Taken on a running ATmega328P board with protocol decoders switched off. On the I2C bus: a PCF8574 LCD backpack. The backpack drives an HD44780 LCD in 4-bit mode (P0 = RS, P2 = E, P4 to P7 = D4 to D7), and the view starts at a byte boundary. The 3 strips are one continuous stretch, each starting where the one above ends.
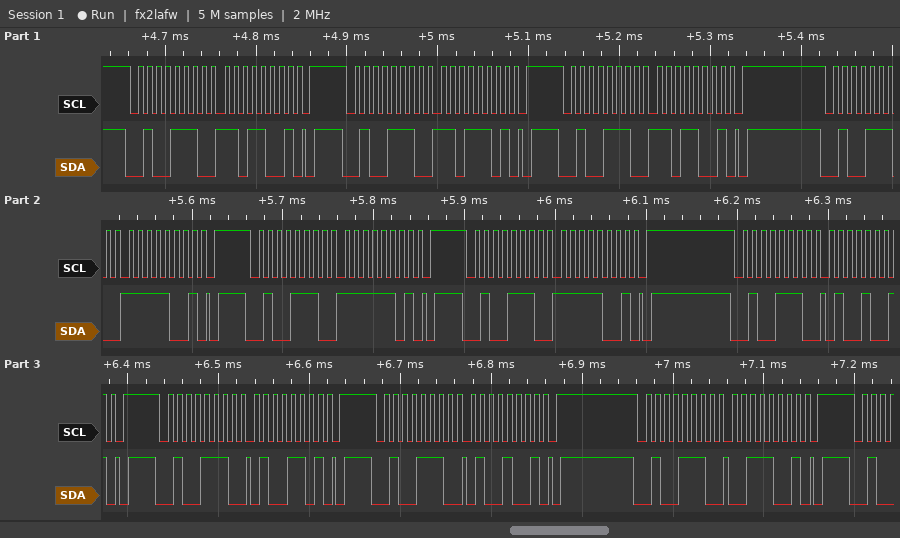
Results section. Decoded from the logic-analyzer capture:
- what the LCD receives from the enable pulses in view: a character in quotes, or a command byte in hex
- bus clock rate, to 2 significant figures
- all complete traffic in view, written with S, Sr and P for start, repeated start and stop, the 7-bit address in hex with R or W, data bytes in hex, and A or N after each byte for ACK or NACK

data 0xDF
100 kHz
S 27W A D9 A P S 27W A DD A P S 27W A D9 A P S 27W A F9 A P S 27W A FD A P S 27W A F9 A P S 27W A 49 A P S 27W A 4D A P S 27W A 49 A P S 27W A 39 A P
